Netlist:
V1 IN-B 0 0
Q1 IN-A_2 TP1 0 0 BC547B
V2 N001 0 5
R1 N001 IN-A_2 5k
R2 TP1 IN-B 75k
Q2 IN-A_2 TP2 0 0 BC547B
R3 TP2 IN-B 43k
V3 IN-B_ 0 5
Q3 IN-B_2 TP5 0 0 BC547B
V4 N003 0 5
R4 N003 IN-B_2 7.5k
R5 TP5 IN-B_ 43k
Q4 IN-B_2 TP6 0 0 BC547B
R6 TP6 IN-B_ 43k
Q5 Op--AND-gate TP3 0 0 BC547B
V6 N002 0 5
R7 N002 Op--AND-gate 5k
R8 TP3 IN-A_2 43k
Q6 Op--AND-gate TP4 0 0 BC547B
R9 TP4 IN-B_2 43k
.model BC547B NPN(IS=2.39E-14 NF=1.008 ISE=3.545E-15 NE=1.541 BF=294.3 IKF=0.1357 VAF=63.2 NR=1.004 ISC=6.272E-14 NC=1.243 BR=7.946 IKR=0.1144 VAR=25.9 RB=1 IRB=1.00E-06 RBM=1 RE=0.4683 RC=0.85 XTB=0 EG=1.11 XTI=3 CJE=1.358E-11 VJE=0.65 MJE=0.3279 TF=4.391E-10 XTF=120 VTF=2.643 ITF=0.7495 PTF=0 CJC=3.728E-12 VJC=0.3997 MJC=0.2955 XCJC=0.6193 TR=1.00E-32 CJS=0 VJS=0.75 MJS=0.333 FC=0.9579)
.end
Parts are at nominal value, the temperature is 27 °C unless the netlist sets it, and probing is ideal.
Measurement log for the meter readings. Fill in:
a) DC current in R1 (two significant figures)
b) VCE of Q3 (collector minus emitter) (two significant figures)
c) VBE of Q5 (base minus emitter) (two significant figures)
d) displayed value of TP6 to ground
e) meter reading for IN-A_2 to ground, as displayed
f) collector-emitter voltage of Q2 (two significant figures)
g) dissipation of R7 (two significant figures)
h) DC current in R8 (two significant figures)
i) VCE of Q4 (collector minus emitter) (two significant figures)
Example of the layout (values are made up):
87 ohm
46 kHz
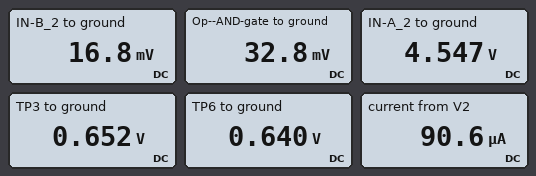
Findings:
91 µA
17 mV
650 mV
0.640 V
4.547 V
4.5 V
4.9 mW
91 µA
17 mV
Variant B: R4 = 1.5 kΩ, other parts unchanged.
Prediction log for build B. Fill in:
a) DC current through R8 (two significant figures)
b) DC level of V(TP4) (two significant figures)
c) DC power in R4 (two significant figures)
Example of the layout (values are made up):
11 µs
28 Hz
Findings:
91 µA
41 mV
16 mW
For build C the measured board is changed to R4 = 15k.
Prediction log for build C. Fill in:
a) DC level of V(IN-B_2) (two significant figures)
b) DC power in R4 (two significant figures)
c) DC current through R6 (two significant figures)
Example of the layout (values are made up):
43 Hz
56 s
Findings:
12 mV
1.7 mW
100 µA
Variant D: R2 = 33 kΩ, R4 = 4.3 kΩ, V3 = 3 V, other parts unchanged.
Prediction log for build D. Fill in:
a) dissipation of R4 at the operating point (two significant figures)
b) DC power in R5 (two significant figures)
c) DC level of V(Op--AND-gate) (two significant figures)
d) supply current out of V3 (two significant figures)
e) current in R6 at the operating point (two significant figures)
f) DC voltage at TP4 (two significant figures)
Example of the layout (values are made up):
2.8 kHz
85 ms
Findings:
5.7 mW
130 µW
33 mV
110 µA
55 µA
32 mV
